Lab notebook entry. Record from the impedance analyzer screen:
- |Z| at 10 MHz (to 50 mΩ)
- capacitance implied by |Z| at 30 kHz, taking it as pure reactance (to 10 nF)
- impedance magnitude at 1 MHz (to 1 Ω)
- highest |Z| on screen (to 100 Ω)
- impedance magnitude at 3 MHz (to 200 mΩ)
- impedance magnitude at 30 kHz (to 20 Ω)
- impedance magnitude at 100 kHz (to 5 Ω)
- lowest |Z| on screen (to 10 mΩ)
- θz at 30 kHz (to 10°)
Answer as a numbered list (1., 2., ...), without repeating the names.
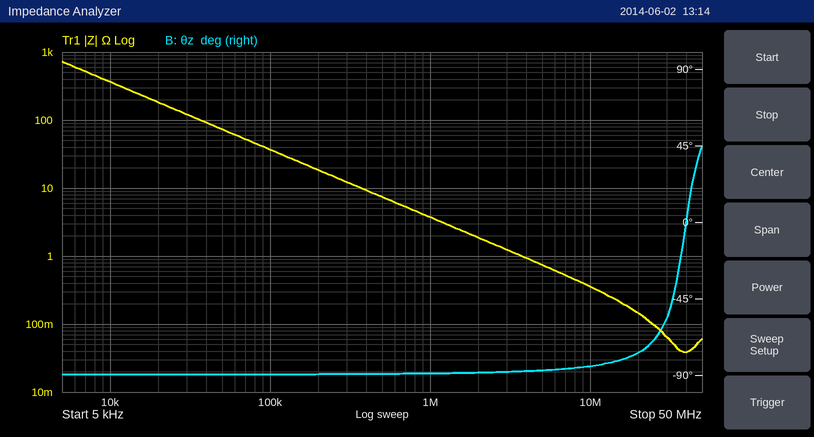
1. 350 mΩ
2. 40 nF
3. 4 Ω
4. 700 Ω
5. 1.2 Ω
6. 120 Ω
7. 35 Ω
8. 40 mΩ
9. -90°
